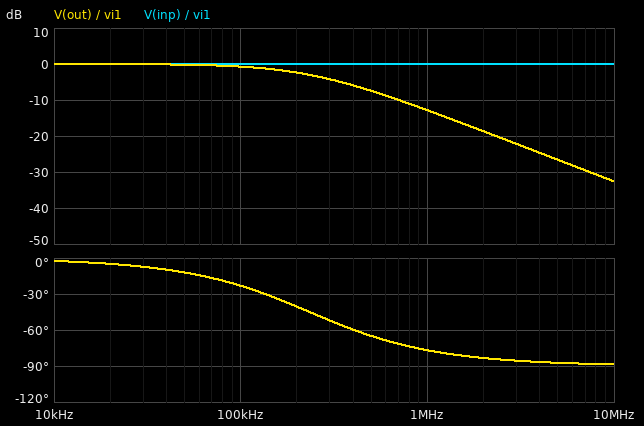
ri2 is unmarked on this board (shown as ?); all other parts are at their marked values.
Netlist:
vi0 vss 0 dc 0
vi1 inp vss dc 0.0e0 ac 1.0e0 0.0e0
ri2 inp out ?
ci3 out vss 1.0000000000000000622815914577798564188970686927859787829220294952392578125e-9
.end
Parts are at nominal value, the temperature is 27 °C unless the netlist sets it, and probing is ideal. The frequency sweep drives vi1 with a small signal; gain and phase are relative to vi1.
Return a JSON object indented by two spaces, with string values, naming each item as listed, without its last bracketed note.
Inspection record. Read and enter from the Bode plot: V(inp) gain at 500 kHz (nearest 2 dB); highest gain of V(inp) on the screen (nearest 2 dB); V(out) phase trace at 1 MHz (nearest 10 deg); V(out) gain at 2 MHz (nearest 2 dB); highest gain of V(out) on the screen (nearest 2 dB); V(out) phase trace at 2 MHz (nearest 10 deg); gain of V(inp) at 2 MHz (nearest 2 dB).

{
  "V(inp) gain at 500 kHz": "0 dB",
  "highest gain of V(inp) on the screen": "0 dB",
  "V(out) phase trace at 1 MHz": "-80 deg",
  "V(out) gain at 2 MHz": "-18 dB",
  "highest gain of V(out) on the screen": "0 dB",
  "V(out) phase trace at 2 MHz": "-80 deg",
  "gain of V(inp) at 2 MHz": "0 dB"
}
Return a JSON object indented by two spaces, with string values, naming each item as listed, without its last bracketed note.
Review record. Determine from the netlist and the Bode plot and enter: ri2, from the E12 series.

{
  "ri2, from the E12 series": "680 Ω"
}
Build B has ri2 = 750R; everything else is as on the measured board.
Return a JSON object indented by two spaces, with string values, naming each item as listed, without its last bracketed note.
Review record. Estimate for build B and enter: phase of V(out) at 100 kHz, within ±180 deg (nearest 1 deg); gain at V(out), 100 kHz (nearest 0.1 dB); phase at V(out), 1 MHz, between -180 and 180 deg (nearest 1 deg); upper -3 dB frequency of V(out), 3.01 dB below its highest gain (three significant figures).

{
  "phase of V(out) at 100 kHz, within ±180 deg": "-25 deg",
  "gain at V(out), 100 kHz": "-0.9 dB",
  "phase at V(out), 1 MHz, between -180 and 180 deg": "-78 deg",
  "upper -3 dB frequency of V(out), 3.01 dB below its highest gain": "212 kHz"
}
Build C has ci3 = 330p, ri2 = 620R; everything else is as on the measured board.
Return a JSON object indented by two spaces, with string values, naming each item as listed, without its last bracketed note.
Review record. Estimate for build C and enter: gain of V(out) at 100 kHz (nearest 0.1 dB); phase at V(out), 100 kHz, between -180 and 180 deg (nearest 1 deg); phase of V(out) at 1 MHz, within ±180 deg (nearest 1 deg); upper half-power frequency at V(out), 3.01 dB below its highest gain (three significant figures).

{
  "gain of V(out) at 100 kHz": "-0.1 dB",
  "phase at V(out), 100 kHz, between -180 and 180 deg": "-7 deg",
  "phase of V(out) at 1 MHz, within ±180 deg": "-52 deg",
  "upper half-power frequency at V(out), 3.01 dB below its highest gain": "778 kHz"
}
